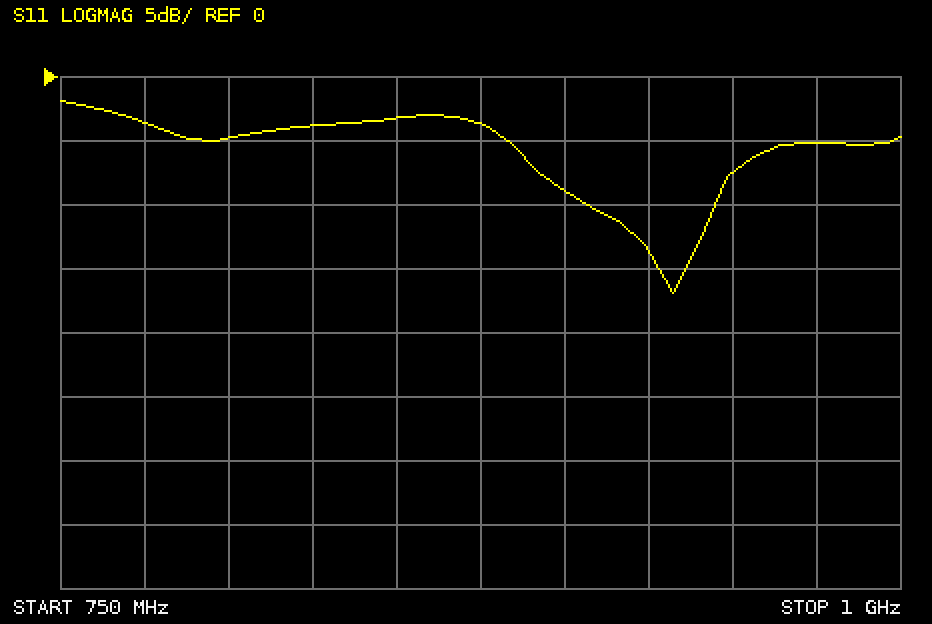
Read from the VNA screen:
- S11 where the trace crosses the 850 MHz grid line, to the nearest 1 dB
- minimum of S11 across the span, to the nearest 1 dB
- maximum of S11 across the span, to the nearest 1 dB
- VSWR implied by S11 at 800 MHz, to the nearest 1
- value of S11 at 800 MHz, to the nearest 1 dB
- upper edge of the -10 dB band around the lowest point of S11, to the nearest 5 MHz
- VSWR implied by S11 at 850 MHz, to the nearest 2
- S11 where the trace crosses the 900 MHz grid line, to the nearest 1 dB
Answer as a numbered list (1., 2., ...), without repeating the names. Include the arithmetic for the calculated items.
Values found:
1. -3 dB
2. -17 dB
3. -2 dB
4. |Γ| = 10^(-5/20) = 0.5623; VSWR = (1 + 0.5623)/(1 − 0.5623) ≈ 4
5. -5 dB
6. 945 MHz
7. |Γ| = 10^(-3/20) = 0.7079; VSWR = (1 + 0.7079)/(1 − 0.7079) ≈ 6
8. -9 dB
